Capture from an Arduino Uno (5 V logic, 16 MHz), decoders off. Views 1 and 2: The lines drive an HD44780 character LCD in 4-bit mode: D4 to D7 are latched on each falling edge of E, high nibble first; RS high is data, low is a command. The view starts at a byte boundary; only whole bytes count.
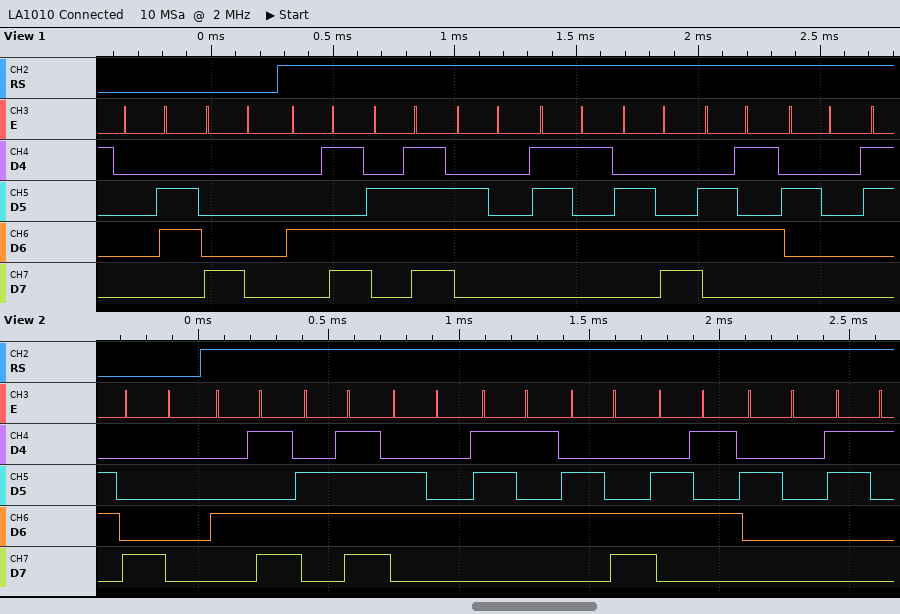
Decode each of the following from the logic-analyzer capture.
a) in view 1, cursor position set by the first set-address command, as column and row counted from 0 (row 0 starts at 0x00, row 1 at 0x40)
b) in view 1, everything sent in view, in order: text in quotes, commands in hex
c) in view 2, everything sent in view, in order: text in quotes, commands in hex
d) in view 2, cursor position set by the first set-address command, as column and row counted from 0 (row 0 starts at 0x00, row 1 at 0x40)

column 0, row 0
0x06 0x80 "Module "
0x80 "Module 1"
column 0, row 0
